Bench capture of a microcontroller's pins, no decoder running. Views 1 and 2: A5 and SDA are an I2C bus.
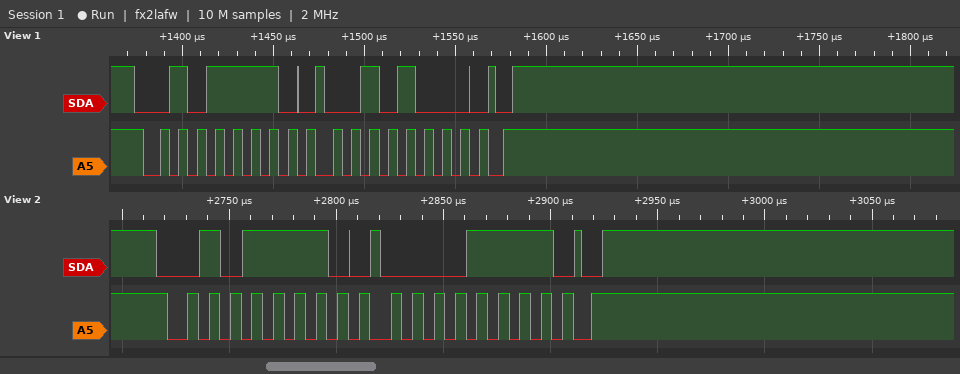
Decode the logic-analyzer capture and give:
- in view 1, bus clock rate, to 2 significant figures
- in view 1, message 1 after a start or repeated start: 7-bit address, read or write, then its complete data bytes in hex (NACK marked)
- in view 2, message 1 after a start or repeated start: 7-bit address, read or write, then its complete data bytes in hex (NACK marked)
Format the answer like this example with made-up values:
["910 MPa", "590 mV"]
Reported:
["100 kHz", "0x2F write: 28", "0x2F write: 0F"]
